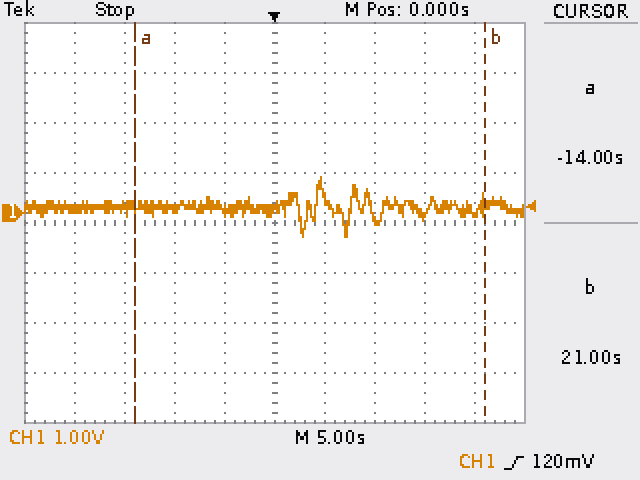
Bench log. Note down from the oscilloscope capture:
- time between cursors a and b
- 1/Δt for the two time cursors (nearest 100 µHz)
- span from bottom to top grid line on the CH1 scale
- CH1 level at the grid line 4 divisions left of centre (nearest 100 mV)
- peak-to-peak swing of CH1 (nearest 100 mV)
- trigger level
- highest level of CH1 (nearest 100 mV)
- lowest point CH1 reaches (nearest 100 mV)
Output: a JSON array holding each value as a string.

["35.0 s", "28.6 mHz", "8 V", "100 mV", "1.2 V", "120 mV", "700 mV", "-500 mV"]
